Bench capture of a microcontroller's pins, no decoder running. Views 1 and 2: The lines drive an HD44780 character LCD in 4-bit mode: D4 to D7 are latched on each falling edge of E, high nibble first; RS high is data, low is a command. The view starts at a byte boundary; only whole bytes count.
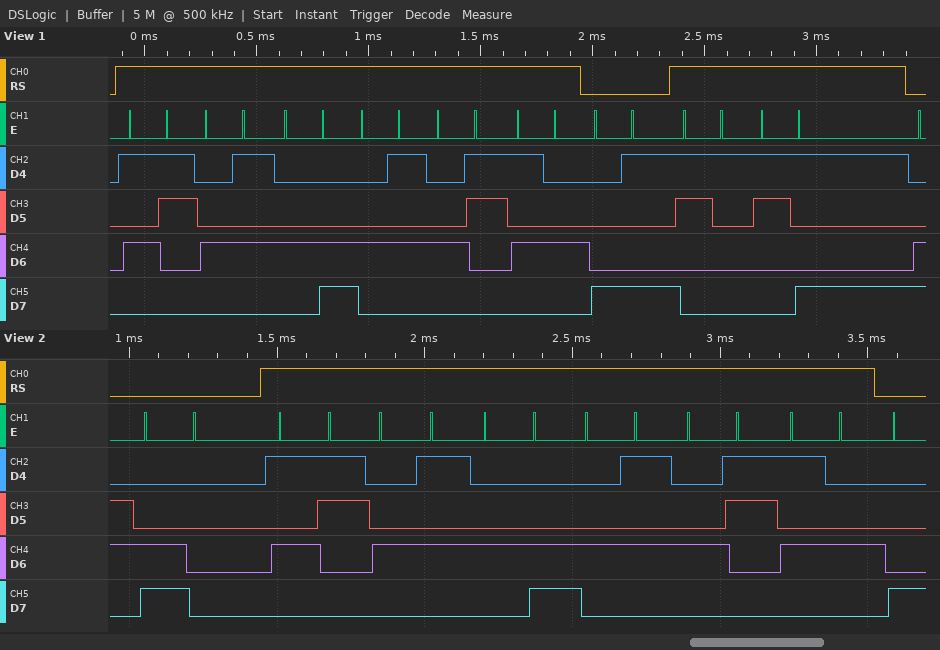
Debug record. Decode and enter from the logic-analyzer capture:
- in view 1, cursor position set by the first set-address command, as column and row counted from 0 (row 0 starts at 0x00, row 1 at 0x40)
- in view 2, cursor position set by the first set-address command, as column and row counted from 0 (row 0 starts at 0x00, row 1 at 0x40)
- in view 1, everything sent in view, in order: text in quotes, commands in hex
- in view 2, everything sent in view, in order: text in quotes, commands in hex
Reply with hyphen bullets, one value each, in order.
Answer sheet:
- column 9, row 0
- column 0, row 1
- "SELECT" 0x89 "19"
- 0xC0 "SELECT"
